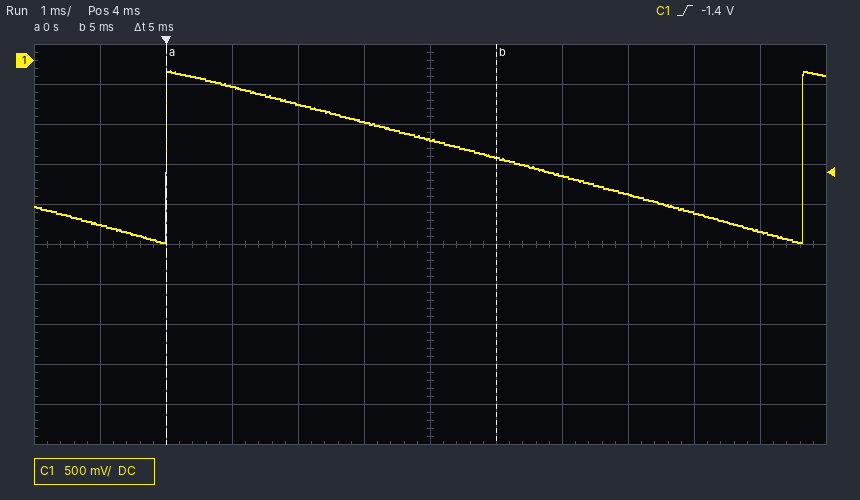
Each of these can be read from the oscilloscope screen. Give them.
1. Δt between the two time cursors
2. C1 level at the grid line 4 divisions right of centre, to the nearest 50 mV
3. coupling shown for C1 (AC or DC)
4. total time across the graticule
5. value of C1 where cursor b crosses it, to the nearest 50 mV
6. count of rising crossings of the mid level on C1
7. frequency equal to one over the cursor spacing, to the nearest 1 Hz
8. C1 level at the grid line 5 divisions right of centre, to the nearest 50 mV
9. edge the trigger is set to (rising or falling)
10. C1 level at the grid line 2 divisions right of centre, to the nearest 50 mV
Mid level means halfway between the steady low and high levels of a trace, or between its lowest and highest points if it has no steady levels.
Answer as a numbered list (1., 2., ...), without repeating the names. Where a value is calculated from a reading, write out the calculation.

1. 5 ms
2. -1.90 V
3. DC
4. 12 ms
5. -1.20 V
6. 2
7. 1 / 5 ms ≈ 200 Hz
8. -2.15 V
9. rising
10. -1.45 V
